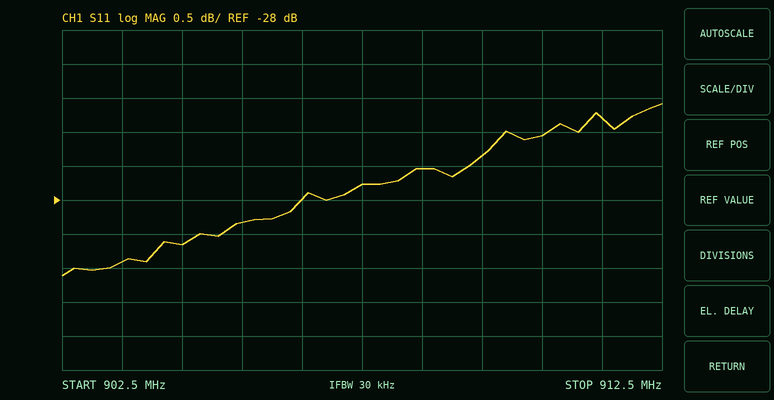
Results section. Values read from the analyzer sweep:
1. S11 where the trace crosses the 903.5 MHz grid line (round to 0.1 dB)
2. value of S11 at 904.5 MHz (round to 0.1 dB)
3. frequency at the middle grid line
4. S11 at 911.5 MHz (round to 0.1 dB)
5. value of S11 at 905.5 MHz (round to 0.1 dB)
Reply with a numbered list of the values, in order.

1. -28.9 dB
2. -28.7 dB
3. 907.5 MHz
4. -26.8 dB
5. -28.3 dB
